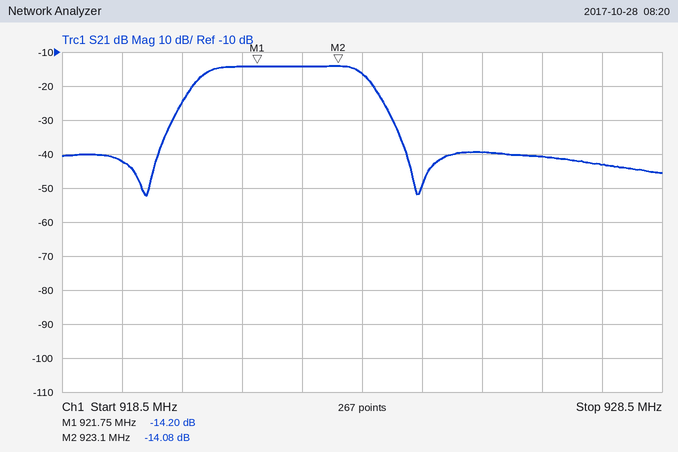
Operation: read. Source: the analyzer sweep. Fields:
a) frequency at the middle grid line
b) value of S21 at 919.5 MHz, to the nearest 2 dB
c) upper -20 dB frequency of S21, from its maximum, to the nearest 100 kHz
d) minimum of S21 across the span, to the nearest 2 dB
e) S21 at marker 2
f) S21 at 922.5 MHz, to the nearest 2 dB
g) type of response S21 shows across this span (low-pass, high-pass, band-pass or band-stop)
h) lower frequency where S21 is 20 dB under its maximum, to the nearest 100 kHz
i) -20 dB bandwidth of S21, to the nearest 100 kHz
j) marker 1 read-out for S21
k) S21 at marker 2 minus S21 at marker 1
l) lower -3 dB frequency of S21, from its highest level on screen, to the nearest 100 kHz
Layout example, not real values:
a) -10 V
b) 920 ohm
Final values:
a) 923.5 MHz
b) -42 dB
c) 924.1 MHz
d) -52 dB
e) -14.08 dB
f) -14 dB
g) band-pass
h) 920.2 MHz
i) 3.9 MHz
j) -14.20 dB
k) 0.12 dB
l) 920.8 MHz
